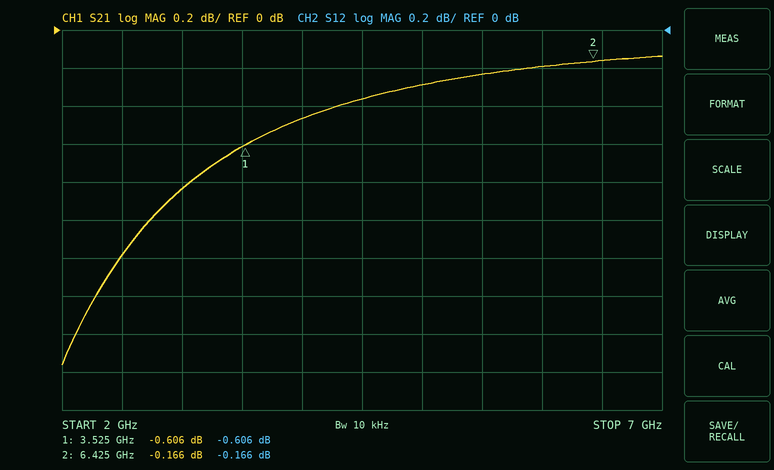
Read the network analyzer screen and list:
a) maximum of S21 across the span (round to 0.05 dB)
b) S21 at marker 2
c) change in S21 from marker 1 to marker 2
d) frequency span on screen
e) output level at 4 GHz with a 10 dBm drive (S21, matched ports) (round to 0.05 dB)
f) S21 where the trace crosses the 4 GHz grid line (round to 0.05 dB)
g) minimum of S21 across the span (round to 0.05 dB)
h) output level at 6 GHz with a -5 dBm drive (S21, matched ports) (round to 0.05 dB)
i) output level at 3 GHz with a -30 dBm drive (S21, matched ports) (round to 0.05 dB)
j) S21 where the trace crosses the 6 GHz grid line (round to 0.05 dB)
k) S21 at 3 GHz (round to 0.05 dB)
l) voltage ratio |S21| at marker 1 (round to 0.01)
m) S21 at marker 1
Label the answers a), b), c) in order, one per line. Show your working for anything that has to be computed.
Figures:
a) -0.15 dB
b) -0.166 dB
c) -0.166 − (-0.606) = 0.440 dB
d) 5 GHz
e) 10 dBm + (-0.45 dB) = 9.55 dBm
f) -0.45 dB
g) -1.75 dB
h) -5 dBm + (-0.20 dB) = -5.20 dBm
i) -30 dBm + (-0.85 dB) = -30.85 dBm
j) -0.20 dB
k) -0.85 dB
l) 10^(-0.606/20) ≈ 0.93
m) -0.606 dB
